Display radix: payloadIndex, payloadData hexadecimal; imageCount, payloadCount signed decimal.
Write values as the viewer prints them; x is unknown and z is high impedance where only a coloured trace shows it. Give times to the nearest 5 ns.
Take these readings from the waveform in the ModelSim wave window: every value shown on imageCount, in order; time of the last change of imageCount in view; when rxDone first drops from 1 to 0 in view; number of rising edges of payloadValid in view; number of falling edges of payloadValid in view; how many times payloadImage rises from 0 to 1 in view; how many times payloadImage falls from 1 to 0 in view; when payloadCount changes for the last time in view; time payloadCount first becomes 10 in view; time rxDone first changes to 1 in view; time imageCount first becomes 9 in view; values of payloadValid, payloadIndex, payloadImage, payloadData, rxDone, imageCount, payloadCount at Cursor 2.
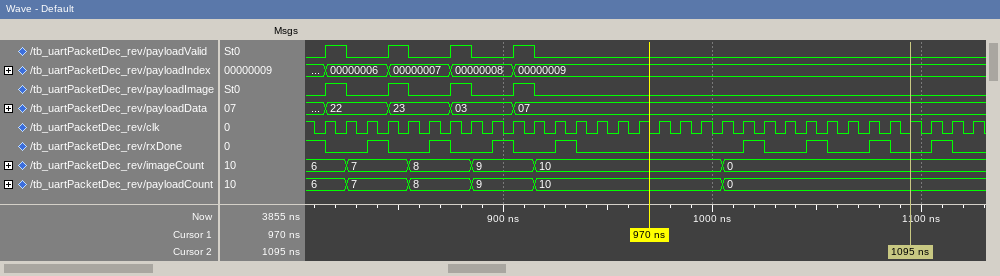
6, 7, 8, 9, 10, 0
1005 ns
815 ns
4
4
4
4
1005 ns
915 ns
835 ns
885 ns
payloadValid=0, payloadIndex=00000009, payloadImage=0, payloadData=07, rxDone=0, imageCount=0, payloadCount=0
